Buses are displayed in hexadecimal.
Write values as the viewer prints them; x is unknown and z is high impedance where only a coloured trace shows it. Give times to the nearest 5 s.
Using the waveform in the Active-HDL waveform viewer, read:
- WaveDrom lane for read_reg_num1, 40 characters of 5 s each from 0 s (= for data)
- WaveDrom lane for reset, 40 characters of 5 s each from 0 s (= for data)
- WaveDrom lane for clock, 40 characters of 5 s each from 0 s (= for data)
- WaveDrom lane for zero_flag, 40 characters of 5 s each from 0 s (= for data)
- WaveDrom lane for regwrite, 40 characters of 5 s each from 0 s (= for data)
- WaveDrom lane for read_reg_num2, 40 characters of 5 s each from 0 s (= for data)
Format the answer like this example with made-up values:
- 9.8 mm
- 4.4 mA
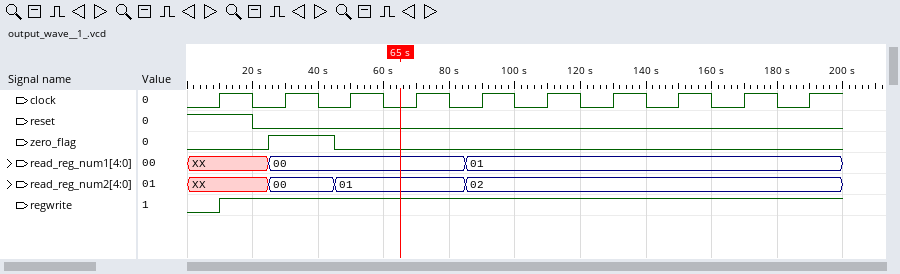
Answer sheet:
- {name: 'read_reg_num1', wave: 'x....=...........=......................', data: '00 01'}
- {name: 'reset', wave: '1...0...................................'}
- {name: 'clock', wave: '0.1.0.1.0.1.0.1.0.1.0.1.0.1.0.1.0.1.0.1.'}
- {name: 'zero_flag', wave: '0....1...0..............................'}
- {name: 'regwrite', wave: '0.1.....................................'}
- {name: 'read_reg_num2', wave: 'x....=...=.......=......................', data: '00 01 02'}
